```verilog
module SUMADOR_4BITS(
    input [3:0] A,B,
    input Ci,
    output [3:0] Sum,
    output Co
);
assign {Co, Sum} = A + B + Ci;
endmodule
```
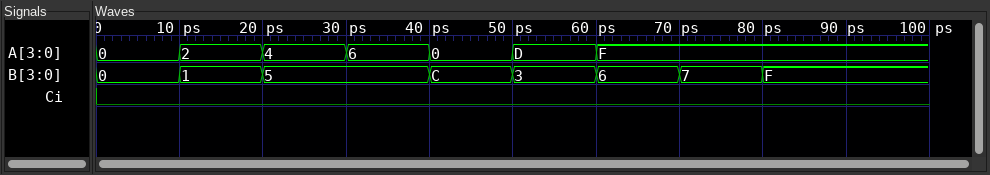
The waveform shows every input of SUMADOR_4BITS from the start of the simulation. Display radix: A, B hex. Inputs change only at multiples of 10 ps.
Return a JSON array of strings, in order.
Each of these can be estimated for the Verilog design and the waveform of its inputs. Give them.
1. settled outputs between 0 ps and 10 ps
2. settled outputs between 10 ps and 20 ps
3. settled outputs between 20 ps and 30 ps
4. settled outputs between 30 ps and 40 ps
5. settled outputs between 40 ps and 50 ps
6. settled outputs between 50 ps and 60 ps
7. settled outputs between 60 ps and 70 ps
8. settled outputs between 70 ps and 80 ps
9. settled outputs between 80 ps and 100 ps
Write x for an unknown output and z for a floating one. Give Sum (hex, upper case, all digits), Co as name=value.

["Sum=0, Co=0", "Sum=3, Co=0", "Sum=9, Co=0", "Sum=B, Co=0", "Sum=C, Co=0", "Sum=0, Co=1", "Sum=5, Co=1", "Sum=6, Co=1", "Sum=E, Co=1"]
